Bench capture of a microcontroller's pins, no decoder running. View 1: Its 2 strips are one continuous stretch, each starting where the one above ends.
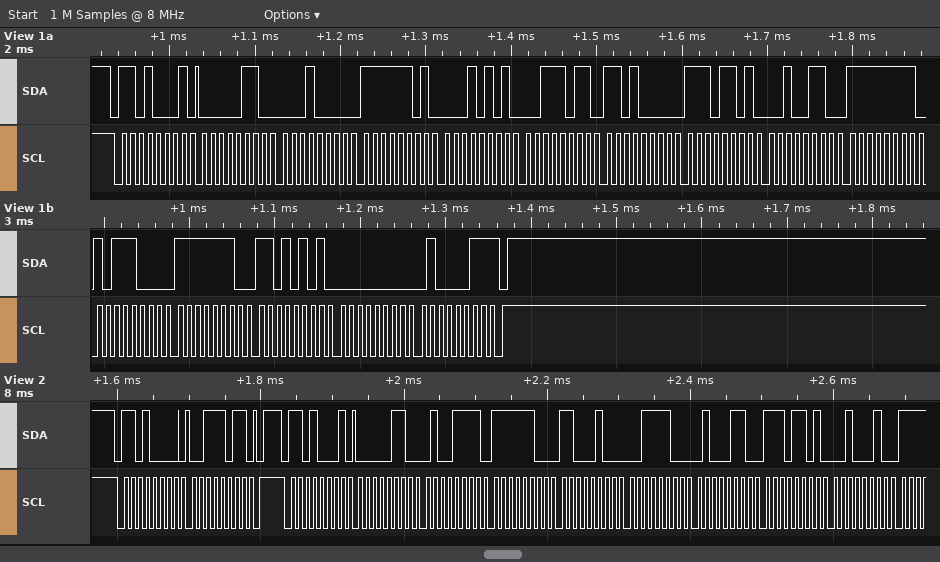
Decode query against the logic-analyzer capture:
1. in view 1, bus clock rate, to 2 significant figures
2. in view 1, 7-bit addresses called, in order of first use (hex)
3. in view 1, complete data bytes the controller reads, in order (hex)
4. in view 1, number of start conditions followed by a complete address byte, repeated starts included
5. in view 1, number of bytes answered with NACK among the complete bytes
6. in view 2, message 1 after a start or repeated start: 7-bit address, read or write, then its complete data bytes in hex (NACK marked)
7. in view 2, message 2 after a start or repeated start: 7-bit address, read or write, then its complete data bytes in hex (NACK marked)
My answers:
100 kHz
0x68
06 10 FD 15 3B D0 ED 26 FF B8 FE D5 00 43
1
1
0x68 write: 3B
0x68 read: 06 4F FC C4 3C 46 ED 22
